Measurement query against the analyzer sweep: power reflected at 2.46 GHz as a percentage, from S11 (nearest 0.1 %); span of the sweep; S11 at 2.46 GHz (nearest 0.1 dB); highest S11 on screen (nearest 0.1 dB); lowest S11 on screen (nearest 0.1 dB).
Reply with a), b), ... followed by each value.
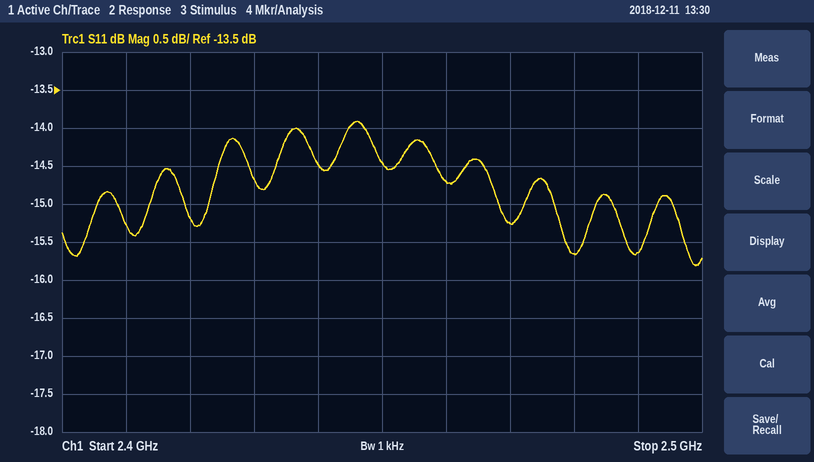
a) 3.4 %
b) 100 MHz
c) -14.7 dB
d) -13.9 dB
e) -15.8 dB
